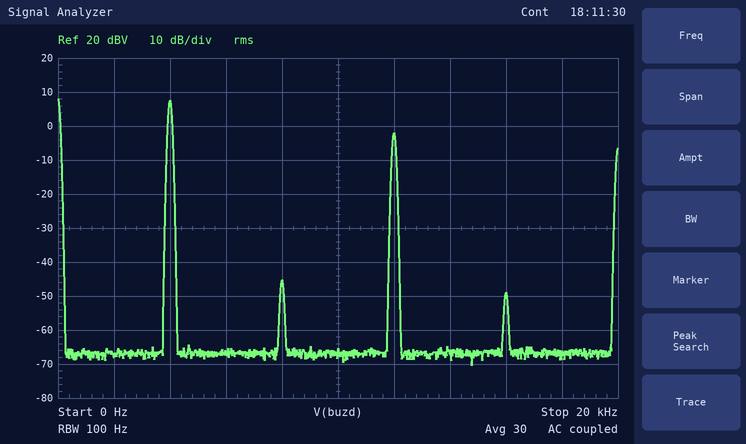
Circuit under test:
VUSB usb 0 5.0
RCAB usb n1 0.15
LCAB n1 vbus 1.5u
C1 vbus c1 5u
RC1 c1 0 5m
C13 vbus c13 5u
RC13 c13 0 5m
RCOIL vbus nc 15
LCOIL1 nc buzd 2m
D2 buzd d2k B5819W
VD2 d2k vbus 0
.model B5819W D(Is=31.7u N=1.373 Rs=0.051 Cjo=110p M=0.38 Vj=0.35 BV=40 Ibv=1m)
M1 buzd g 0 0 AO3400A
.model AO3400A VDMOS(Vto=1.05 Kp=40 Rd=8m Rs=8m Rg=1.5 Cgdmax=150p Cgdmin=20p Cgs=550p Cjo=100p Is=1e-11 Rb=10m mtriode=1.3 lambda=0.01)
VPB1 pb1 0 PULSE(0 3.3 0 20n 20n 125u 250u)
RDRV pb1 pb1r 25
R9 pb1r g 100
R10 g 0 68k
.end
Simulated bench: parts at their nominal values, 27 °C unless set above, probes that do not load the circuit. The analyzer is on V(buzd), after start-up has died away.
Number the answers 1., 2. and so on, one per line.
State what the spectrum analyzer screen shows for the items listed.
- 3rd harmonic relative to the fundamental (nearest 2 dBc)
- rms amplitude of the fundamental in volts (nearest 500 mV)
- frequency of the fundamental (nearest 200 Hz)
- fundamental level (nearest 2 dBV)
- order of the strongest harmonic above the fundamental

1. -10 dBc
2. 2.5 V
3. 4.0 kHz
4. 8 dBV
5. 3
